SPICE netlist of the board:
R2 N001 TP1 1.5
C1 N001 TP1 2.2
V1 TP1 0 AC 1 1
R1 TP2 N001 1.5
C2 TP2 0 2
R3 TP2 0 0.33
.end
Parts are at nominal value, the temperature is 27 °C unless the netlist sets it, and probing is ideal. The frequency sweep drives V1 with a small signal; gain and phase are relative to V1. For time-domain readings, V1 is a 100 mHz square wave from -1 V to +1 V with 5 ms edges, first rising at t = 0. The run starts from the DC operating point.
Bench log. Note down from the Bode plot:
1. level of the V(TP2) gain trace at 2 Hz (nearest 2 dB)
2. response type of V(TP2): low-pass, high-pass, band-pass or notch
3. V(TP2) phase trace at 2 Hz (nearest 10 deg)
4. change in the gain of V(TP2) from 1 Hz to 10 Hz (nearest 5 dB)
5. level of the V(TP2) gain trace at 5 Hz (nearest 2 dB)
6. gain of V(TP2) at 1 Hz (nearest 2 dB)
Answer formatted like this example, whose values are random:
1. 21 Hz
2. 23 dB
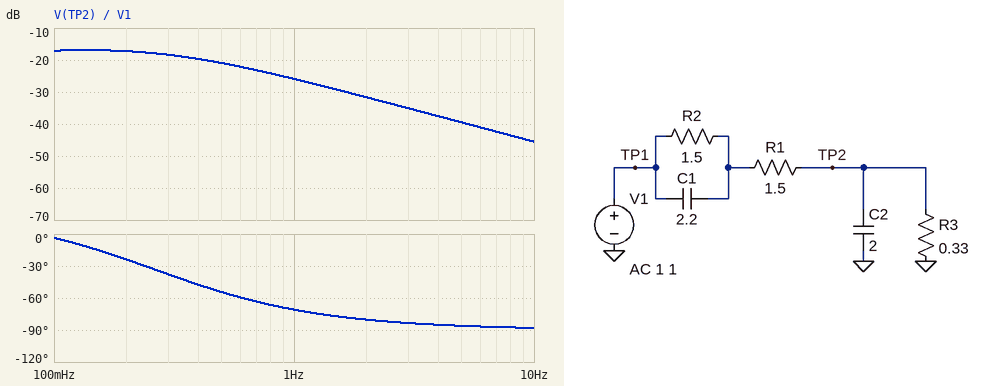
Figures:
1. -32 dB
2. low-pass
3. -80 deg
4. -20 dB
5. -40 dB
6. -26 dB
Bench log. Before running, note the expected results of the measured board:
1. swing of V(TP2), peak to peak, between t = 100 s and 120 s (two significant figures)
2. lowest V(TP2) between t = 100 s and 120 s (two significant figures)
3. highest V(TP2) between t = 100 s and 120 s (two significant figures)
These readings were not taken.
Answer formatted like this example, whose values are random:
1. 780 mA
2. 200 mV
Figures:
1. 330 mV
2. -160 mV
3. 160 mV
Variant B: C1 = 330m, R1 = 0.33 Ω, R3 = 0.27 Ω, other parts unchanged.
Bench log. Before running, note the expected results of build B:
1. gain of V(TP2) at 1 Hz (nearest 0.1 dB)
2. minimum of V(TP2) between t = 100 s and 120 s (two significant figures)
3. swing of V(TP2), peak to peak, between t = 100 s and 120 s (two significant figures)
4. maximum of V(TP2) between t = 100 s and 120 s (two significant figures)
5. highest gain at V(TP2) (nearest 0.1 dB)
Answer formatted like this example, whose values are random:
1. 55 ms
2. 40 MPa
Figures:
1. -19.4 dB
2. -130 mV
3. 260 mV
4. 130 mV
5. -17.8 dB
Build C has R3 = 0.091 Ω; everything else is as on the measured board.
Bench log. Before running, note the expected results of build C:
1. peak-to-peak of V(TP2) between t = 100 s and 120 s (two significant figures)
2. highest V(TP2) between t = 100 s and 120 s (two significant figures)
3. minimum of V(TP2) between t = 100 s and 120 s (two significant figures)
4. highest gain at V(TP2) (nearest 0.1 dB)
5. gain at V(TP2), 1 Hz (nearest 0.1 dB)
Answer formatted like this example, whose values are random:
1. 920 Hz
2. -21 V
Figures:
1. 130 mV
2. 67 mV
3. -67 mV
4. -25.6 dB
5. -28.2 dB
